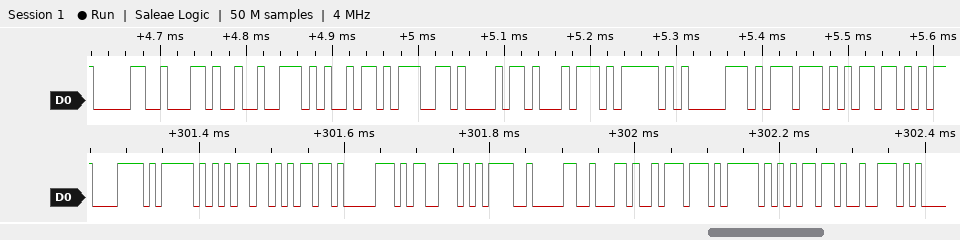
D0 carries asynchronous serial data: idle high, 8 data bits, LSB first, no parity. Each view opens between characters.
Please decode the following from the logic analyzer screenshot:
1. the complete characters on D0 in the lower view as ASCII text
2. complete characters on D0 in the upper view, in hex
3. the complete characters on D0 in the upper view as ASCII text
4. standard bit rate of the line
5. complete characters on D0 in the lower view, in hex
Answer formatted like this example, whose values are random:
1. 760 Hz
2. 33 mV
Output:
1. "x_mmps=0,w_mr"
2. 30, 2C, 72, 69, 67, 68, 74, 5F, 70, 77, 6D
3. "0,right_pwm"
4. 115200 baud
5. 78, 5F, 6D, 6D, 70, 73, 3D, 30, 2C, 77, 5F, 6D, 72
